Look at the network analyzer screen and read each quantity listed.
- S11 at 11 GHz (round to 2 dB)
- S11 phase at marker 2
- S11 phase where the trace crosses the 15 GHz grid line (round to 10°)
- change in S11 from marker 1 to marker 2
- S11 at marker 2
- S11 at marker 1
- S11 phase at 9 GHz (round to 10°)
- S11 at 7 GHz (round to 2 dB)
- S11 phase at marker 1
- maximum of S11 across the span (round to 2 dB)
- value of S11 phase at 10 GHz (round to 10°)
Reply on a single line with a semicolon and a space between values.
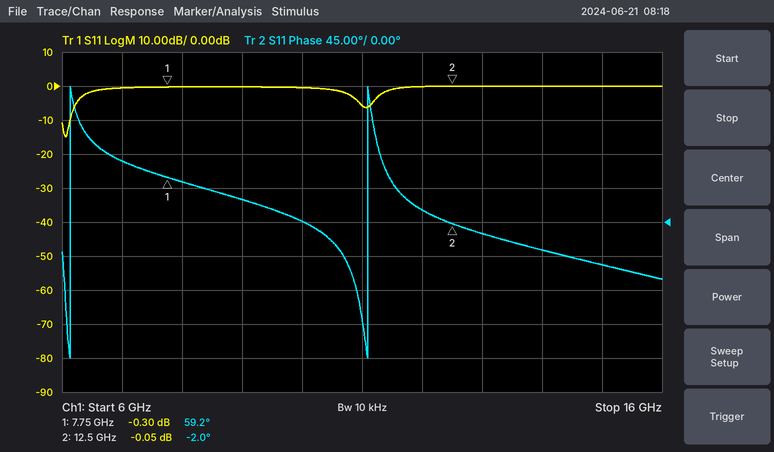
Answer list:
-6 dB; -2.0°; -60°; 0.25 dB; -0.05 dB; -0.30 dB; 30°; 0 dB; 59.2°; 0 dB; 0°
